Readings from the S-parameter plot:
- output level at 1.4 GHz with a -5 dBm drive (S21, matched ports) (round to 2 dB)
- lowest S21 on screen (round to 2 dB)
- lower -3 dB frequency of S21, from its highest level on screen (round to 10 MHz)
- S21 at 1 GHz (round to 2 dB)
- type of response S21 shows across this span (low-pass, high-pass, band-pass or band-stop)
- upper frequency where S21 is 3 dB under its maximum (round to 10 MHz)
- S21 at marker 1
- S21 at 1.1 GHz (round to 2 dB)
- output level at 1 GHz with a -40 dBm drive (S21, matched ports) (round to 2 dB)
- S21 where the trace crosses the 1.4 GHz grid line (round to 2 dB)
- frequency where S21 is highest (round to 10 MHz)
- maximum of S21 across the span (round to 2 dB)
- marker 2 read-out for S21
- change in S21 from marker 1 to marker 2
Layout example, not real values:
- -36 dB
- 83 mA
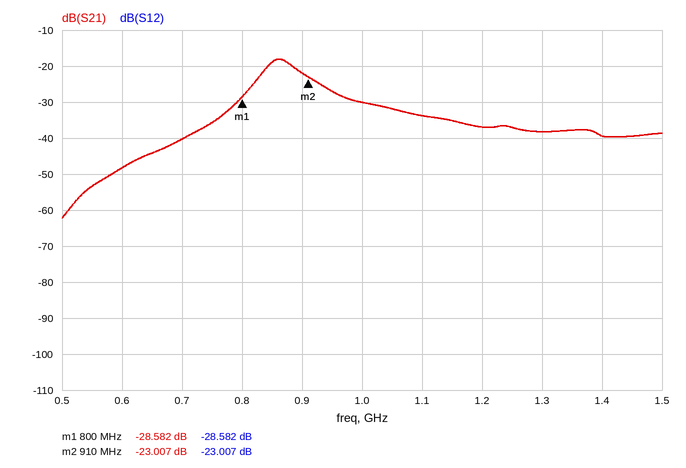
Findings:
- -44 dBm
- -62 dB
- 840 MHz
- -30 dB
- band-pass
- 890 MHz
- -28.582 dB
- -34 dB
- -70 dBm
- -40 dB
- 860 MHz
- -18 dB
- -23.007 dB
- 5.575 dB
